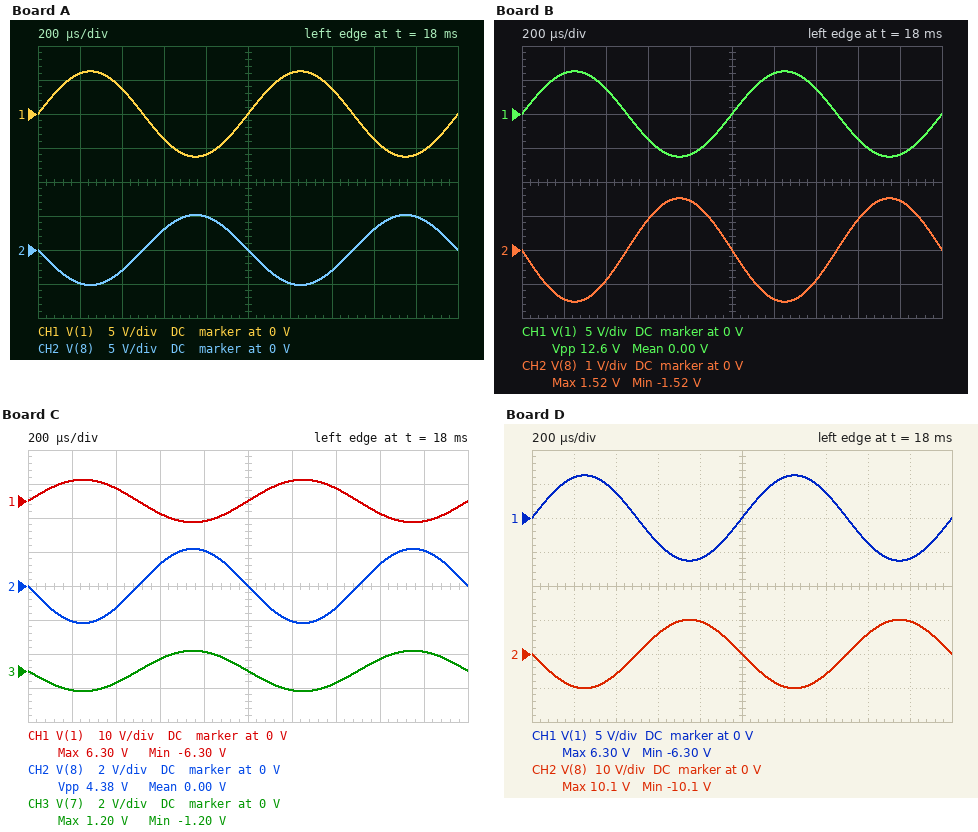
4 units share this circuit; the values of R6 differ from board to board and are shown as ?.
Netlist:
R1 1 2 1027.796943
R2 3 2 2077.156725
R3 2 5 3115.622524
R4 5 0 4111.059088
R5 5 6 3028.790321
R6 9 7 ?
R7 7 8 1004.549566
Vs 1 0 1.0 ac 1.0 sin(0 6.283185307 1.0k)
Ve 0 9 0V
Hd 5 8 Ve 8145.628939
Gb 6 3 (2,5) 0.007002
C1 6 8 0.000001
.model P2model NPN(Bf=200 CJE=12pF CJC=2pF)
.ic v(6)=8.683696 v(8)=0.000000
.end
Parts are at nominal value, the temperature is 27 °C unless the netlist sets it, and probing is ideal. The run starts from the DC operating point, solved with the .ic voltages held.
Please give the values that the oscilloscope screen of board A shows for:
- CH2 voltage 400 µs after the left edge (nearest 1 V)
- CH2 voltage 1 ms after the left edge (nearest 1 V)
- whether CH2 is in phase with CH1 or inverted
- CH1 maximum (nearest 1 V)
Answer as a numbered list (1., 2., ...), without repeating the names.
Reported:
1. -3 V
2. 0 V
3. inverted
4. 6 V
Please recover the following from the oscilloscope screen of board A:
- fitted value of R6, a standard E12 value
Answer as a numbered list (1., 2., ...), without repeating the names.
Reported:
1. 2.7 kΩ
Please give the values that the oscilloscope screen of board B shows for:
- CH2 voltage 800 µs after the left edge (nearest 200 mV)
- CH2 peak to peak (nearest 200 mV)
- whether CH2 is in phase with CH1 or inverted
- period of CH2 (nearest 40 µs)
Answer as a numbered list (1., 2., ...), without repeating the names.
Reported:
1. 1.4 V
2. 3.0 V
3. inverted
4. 1.00 ms
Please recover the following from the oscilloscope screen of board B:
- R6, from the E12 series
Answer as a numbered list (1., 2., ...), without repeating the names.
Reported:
1. 680 Ω
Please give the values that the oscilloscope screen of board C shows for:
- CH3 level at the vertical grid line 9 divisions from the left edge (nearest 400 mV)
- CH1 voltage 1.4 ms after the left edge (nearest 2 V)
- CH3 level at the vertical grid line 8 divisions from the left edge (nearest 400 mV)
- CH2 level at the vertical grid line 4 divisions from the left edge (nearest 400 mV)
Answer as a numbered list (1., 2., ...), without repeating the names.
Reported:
1. 1.2 V
2. 4 V
3. 800 mV
4. 2.0 V
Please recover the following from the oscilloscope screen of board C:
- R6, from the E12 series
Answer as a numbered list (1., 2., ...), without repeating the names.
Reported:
1. 1.2 kΩ
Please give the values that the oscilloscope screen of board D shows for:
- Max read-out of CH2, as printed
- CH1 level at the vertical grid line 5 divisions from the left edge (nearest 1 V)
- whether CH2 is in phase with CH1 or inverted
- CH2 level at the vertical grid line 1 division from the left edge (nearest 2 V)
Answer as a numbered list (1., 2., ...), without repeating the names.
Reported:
1. 10.1 V
2. 0 V
3. inverted
4. -10 V
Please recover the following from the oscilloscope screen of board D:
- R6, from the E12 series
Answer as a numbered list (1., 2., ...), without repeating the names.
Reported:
1. 3.9 kΩ
